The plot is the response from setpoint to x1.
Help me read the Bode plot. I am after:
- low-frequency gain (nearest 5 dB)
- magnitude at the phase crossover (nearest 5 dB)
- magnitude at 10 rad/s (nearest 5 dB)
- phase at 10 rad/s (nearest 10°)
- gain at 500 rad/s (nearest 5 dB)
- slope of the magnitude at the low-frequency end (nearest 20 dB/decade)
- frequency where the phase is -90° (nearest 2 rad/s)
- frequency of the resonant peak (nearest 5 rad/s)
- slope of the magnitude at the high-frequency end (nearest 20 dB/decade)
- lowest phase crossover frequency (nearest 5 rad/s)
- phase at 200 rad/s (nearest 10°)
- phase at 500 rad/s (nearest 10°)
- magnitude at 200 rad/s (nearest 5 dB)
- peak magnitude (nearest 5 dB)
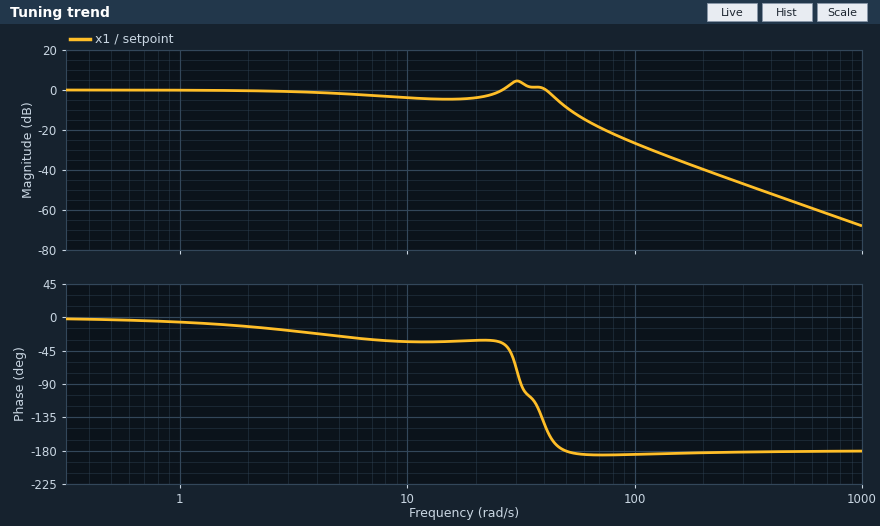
0 dB
-10 dB
-5 dB
-30°
-55 dB
0 dB/decade
32 rad/s
30 rad/s
-40 dB/decade
50 rad/s
-180°
-180°
-40 dB
5 dB
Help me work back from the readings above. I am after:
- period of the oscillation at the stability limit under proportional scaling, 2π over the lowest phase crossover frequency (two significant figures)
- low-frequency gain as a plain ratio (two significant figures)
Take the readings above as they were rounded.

0.13 s
1.0
